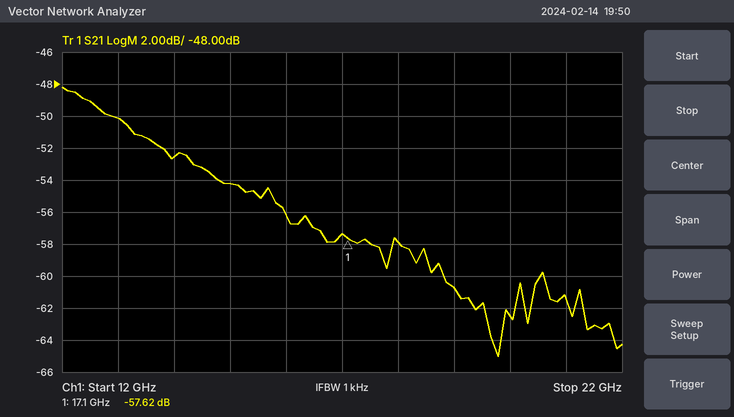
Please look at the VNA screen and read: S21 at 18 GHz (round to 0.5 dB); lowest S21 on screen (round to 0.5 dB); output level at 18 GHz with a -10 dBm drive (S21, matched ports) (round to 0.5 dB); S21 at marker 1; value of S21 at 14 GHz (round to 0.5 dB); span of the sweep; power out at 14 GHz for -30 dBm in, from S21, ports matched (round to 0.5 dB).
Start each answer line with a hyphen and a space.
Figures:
- -58.0 dB
- -65.0 dB
- -68.0 dBm
- -57.62 dB
- -52.5 dB
- 10 GHz
- -82.5 dBm
